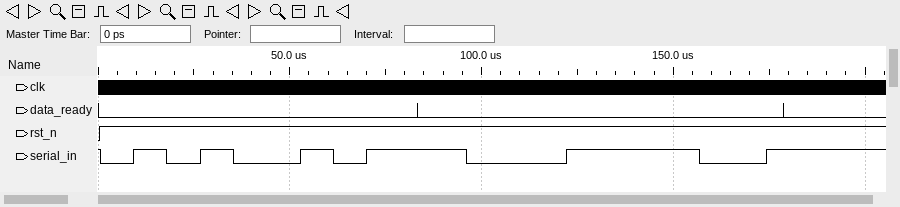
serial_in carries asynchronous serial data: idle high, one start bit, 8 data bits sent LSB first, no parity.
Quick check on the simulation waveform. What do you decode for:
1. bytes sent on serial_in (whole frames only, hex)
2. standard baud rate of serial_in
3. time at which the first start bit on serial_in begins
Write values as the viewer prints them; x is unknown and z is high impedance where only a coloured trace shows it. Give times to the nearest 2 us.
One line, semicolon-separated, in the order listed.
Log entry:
A5, 3C; 115200 baud; 0 us
